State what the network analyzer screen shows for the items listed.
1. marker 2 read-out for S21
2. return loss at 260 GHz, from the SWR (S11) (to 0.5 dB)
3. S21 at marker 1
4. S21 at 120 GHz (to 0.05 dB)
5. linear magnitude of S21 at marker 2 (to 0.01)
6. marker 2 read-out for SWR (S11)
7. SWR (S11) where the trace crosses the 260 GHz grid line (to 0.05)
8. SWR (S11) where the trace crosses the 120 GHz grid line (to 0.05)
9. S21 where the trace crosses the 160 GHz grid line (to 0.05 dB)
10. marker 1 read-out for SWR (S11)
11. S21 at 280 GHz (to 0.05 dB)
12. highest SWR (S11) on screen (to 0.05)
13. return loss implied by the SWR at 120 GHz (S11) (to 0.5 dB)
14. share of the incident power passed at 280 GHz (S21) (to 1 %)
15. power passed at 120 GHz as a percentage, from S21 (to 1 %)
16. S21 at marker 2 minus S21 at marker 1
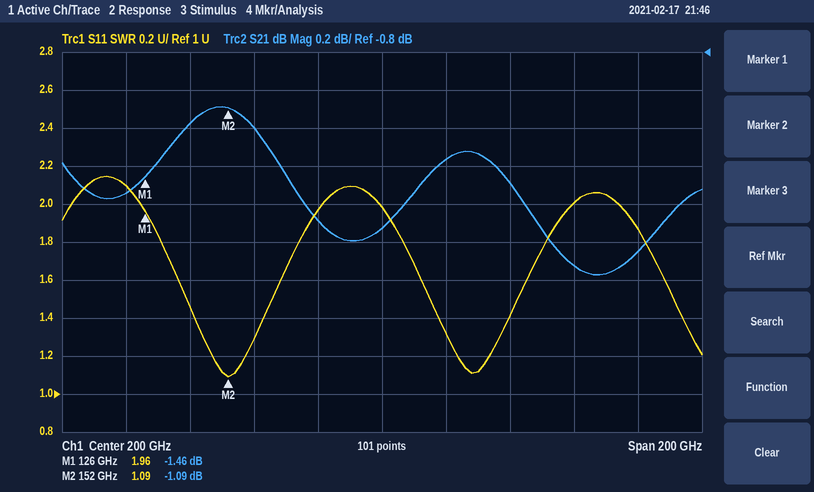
-1.09 dB
9.5 dB
-1.46 dB
-1.55 dB
0.88
1.09
2.00
2.10
-1.20 dB
1.96
-1.85 dB
2.15
9.0 dB
65 %
70 %
0.37 dB
